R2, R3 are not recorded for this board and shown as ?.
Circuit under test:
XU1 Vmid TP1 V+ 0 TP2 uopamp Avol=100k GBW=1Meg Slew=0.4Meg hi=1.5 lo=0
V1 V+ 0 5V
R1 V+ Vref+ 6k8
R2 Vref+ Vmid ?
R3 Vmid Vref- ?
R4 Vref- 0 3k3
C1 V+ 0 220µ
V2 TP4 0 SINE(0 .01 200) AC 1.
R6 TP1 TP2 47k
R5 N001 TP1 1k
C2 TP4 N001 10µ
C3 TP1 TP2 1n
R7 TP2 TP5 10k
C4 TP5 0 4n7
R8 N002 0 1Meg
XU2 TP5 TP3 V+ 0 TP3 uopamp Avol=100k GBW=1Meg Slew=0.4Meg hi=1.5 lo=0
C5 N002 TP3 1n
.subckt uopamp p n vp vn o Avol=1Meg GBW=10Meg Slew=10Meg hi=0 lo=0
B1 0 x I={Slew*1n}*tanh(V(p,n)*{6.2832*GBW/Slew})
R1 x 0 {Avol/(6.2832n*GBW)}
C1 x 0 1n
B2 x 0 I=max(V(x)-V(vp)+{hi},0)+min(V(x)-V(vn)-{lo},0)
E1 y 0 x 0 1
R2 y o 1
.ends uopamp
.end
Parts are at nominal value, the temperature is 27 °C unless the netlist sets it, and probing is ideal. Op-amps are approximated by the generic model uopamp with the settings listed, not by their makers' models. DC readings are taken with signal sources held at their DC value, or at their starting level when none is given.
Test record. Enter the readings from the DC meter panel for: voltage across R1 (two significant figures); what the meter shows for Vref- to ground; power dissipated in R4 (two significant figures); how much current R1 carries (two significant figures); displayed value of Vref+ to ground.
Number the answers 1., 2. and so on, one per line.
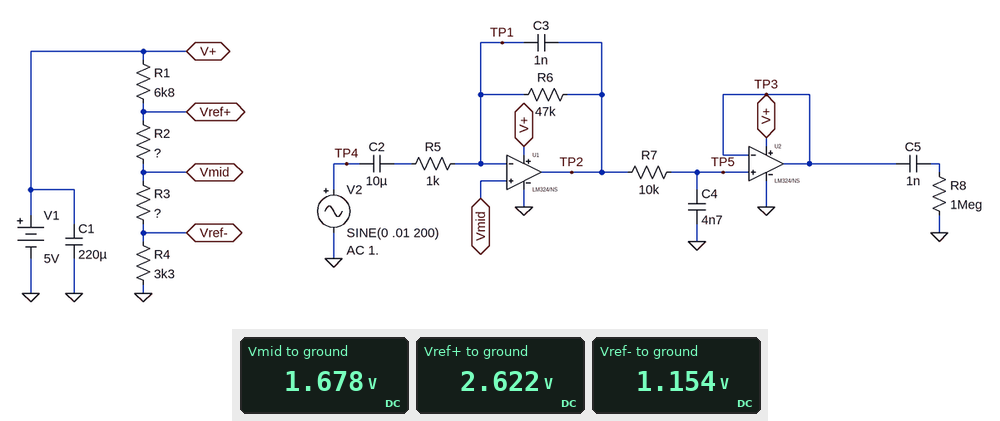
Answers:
1. 2.4 V
2. 1.154 V
3. 400 µW
4. 350 µA
5. 2.622 V
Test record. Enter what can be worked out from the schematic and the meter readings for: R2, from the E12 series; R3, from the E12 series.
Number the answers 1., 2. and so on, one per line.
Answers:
1. 2.7 kΩ
2. 1.5 kΩ
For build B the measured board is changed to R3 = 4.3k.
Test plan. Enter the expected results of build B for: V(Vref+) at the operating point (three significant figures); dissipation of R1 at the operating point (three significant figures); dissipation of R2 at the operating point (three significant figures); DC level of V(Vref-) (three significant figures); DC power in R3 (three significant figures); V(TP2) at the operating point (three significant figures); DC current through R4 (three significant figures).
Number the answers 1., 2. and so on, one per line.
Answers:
1. 3.01 V
2. 581 µW
3. 231 µW
4. 965 mV
5. 368 µW
6. 2.22 V
7. 292 µA
